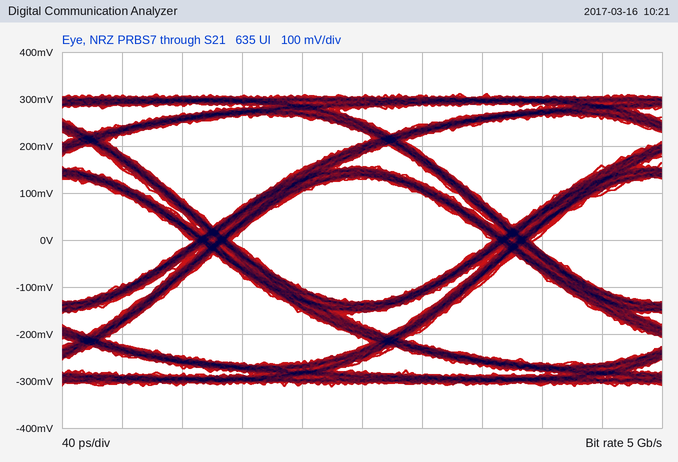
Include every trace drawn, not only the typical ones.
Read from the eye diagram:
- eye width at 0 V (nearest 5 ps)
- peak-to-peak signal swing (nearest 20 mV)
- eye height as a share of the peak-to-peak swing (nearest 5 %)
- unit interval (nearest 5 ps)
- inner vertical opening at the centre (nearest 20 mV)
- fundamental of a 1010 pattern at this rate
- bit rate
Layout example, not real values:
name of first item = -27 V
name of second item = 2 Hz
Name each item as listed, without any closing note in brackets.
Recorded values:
eye width at 0 V = 175 ps
peak-to-peak signal swing = 620 mV
eye height as a share of the peak-to-peak swing = 40 %
unit interval = 200 ps
inner vertical opening at the centre = 260 mV
fundamental of a 1010 pattern at this rate = 2.5 GHz
bit rate = 5 Gb/s
